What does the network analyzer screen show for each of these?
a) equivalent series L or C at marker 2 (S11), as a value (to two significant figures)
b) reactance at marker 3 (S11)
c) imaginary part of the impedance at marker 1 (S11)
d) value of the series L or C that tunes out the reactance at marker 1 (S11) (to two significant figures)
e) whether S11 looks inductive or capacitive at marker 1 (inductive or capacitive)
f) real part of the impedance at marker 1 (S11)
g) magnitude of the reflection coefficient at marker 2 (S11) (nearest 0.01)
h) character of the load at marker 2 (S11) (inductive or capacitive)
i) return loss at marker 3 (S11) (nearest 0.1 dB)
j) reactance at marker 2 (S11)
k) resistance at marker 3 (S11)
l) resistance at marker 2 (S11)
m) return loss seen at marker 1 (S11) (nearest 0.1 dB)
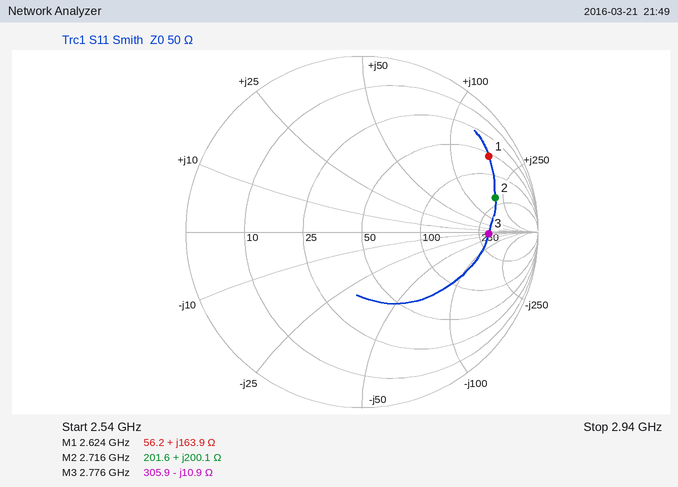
12 nH
-10.9 Ω
+163.9 Ω
370 fF
inductive
56.2 Ω
0.78
inductive
2.9 dB
+200.1 Ω
305.9 Ω
201.6 Ω
1.5 dB
